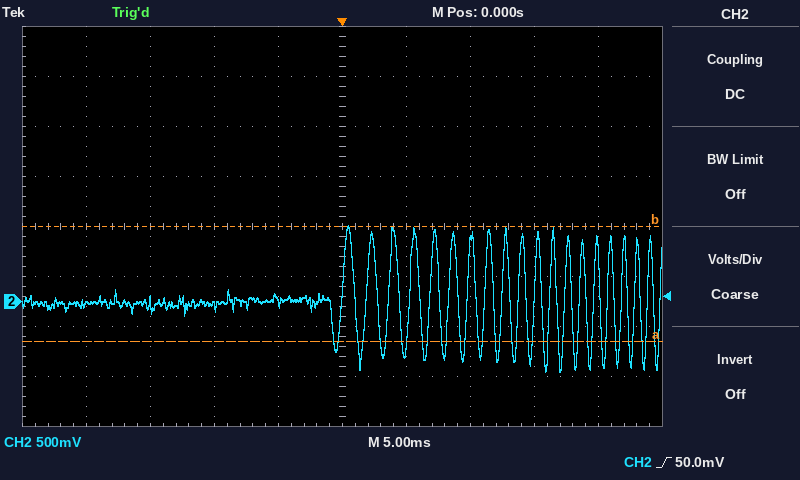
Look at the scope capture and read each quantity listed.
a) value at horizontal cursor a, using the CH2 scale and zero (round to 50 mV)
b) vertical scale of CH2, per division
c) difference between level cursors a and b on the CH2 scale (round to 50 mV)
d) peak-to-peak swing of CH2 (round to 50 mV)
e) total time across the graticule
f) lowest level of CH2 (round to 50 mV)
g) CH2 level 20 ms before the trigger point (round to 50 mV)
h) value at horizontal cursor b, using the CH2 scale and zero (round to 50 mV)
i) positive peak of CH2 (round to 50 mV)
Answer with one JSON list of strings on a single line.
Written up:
["-400 mV", "500 mV", "1.15 V", "1.45 V", "50 ms", "-700 mV", "-50 mV", "750 mV", "750 mV"]
